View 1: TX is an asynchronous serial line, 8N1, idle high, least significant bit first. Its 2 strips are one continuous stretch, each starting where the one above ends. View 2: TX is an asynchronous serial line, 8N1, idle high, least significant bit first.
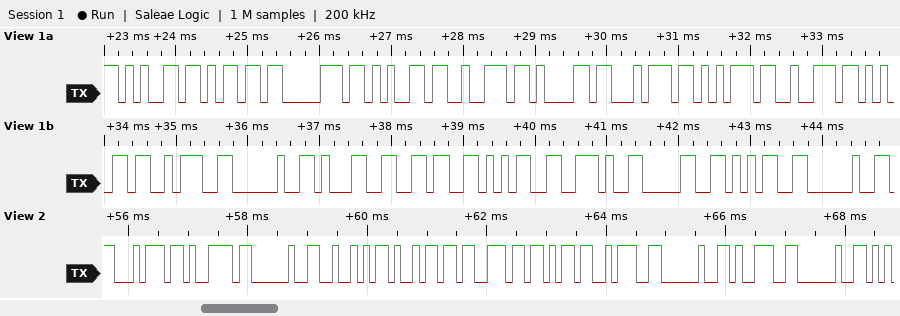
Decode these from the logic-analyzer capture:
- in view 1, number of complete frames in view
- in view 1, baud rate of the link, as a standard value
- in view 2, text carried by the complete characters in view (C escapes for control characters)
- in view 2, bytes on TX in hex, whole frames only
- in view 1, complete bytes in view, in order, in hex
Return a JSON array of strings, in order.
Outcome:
["19", "9600 baud", "\"ty Risk: 9 \"", "74 79 20 52 69 73 6B 3A 20 39 20", "65 6D 70 65 72 61 74 75 72 65 3A 20 31 36 35 2E 30 35 20"]
